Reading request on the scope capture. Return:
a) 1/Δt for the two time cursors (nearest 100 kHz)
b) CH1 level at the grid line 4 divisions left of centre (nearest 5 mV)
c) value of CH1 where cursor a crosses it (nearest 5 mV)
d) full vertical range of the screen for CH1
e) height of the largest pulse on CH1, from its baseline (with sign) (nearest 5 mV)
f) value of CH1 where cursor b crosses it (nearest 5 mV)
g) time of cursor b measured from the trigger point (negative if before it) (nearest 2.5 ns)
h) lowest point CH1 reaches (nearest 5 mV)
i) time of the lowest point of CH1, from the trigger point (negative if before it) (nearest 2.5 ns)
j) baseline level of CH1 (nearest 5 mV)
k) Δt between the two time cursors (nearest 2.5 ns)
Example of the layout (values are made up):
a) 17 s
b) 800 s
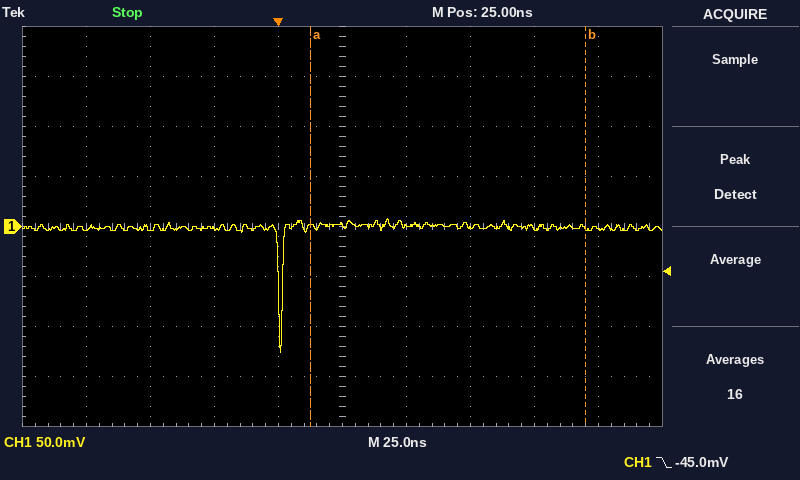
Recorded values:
a) 9.3 MHz
b) -5 mV
c) 0 mV
d) 400 mV
e) -125 mV
f) 0 mV
g) +120.0 ns
h) -125 mV
i) 0.0 ns
j) 0 mV
k) 107.5 ns
